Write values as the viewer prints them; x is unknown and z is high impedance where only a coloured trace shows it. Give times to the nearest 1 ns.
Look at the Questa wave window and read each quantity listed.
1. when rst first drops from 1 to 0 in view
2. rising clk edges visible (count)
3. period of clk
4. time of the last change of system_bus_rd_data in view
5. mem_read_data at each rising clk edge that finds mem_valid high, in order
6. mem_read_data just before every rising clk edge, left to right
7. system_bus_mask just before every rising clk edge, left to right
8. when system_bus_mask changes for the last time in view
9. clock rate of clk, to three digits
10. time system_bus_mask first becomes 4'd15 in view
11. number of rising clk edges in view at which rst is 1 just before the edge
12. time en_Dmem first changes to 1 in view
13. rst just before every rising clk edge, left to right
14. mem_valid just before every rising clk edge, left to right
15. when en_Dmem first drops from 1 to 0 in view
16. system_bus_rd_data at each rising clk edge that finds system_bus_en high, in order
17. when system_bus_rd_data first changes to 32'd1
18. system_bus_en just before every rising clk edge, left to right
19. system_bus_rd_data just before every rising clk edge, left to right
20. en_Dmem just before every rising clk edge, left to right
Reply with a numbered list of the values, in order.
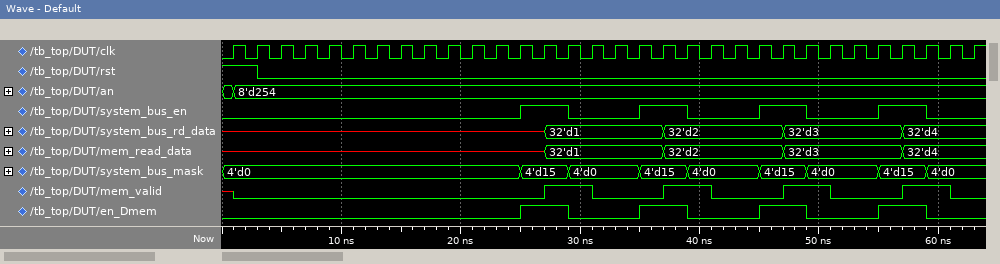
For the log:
1. 3 ns
2. 32
3. 2 ns
4. 57 ns
5. 32'd1, 32'd1, 32'd2, 32'd2, 32'd3, 32'd3, 32'd4, 32'd4
6. x, x, x, x, x, x, x, x, x, x, x, x, x, x, 32'd1, 32'd1, 32'd1, 32'd1, 32'd1, 32'd2, 32'd2, 32'd2, 32'd2, 32'd2, 32'd3, 32'd3, 32'd3, 32'd3, 32'd3, 32'd4, 32'd4, 32'd4
7. 4'd0, 4'd0, 4'd0, 4'd0, 4'd0, 4'd0, 4'd0, 4'd0, 4'd0, 4'd0, 4'd0, 4'd0, 4'd0, 4'd15, 4'd15, 4'd0, 4'd0, 4'd0, 4'd15, 4'd15, 4'd0, 4'd0, 4'd0, 4'd15, 4'd15, 4'd0, 4'd0, 4'd0, 4'd15, 4'd15, 4'd0, 4'd0
8. 59 ns
9. 500 MHz
10. 25 ns
11. 2
12. 25 ns
13. 1 1 0 0 0 0 0 0 0 0 0 0 0 0 0 0 0 0 0 0 0 0 0 0 0 0 0 0 0 0 0 0
14. x 0 0 0 0 0 0 0 0 0 0 0 0 0 1 1 0 0 0 1 1 0 0 0 1 1 0 0 0 1 1 0
15. 29 ns
16. x, 32'd1, 32'd1, 32'd2, 32'd2, 32'd3, 32'd3, 32'd4
17. 27 ns
18. 0 0 0 0 0 0 0 0 0 0 0 0 0 1 1 0 0 0 1 1 0 0 0 1 1 0 0 0 1 1 0 0
19. x, x, x, x, x, x, x, x, x, x, x, x, x, x, 32'd1, 32'd1, 32'd1, 32'd1, 32'd1, 32'd2, 32'd2, 32'd2, 32'd2, 32'd2, 32'd3, 32'd3, 32'd3, 32'd3, 32'd3, 32'd4, 32'd4, 32'd4
20. 0 0 0 0 0 0 0 0 0 0 0 0 0 1 1 0 0 0 1 1 0 0 0 1 1 0 0 0 1 1 0 0
